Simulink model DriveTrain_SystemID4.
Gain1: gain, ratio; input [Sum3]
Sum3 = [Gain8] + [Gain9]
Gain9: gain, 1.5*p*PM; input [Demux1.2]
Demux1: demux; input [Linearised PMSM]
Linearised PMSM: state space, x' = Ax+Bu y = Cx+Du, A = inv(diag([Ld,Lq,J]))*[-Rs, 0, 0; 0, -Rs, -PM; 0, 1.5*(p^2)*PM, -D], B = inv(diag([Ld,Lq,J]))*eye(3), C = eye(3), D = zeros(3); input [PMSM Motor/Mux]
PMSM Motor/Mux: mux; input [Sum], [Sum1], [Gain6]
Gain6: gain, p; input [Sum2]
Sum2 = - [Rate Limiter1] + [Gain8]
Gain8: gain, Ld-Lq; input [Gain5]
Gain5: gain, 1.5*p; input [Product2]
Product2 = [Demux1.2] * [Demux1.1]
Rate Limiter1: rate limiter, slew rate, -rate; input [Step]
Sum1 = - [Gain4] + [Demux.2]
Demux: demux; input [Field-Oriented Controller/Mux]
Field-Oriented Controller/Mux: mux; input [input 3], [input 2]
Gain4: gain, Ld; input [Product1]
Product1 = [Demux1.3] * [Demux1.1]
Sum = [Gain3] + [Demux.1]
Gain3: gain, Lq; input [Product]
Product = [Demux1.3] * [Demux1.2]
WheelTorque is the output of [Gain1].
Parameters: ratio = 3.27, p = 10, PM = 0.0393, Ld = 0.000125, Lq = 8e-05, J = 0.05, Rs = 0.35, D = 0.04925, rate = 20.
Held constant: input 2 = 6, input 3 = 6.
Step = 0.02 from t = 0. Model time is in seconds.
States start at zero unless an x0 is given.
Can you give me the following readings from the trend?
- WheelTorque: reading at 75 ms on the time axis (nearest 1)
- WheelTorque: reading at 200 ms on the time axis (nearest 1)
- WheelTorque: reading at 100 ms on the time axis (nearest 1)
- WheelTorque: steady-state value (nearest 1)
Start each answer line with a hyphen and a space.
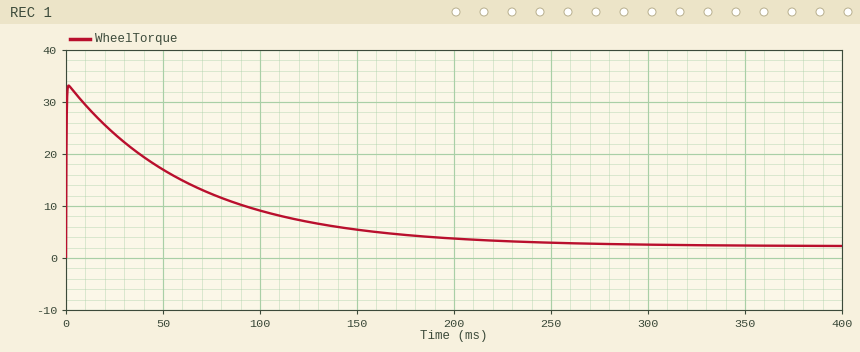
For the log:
- 12
- 4
- 9
- 2
